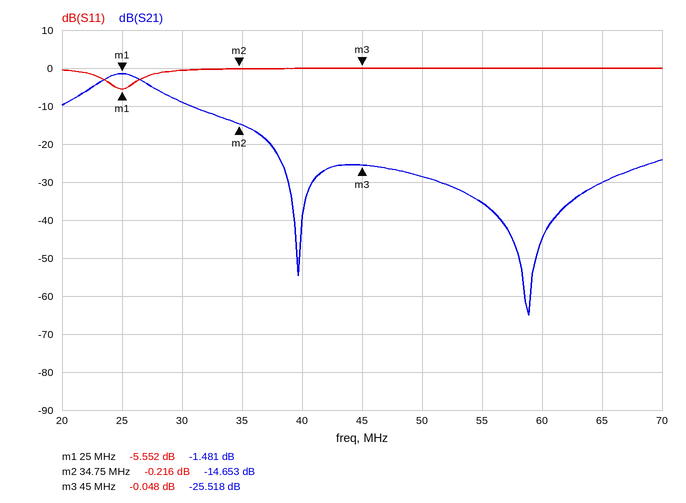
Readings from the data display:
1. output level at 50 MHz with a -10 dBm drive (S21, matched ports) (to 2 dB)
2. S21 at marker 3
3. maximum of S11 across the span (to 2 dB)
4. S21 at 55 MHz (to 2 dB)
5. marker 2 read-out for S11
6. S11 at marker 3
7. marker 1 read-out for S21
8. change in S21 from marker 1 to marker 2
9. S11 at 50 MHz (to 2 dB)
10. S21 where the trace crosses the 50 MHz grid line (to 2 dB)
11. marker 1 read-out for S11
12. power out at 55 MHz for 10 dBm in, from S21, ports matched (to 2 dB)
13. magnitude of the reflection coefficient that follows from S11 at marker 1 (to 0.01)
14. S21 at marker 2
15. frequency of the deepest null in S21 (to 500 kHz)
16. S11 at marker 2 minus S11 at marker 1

-38 dBm
-25.518 dB
0 dB
-36 dB
-0.216 dB
-0.048 dB
-1.481 dB
-13.172 dB
0 dB
-28 dB
-5.552 dB
-26 dBm
0.53
-14.653 dB
59.0 MHz
5.336 dB
